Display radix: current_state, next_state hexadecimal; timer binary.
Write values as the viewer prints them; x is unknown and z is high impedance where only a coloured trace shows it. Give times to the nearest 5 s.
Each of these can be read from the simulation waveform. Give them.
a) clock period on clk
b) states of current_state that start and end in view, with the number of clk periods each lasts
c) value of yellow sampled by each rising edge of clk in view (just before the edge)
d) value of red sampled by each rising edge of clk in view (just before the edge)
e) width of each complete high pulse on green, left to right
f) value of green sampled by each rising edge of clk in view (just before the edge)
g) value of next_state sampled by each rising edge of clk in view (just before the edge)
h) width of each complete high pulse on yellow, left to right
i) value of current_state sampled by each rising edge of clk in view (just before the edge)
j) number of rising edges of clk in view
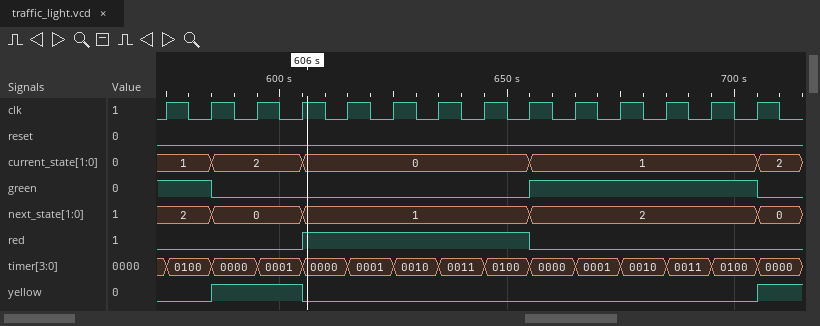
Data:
10 s
2: 2, 0: 5, 1: 5
0 0 1 1 0 0 0 0 0 0 0 0 0 0
0 0 0 0 1 1 1 1 1 0 0 0 0 0
50 s
1 1 0 0 0 0 0 0 0 1 1 1 1 1
2, 2, 0, 0, 1, 1, 1, 1, 1, 2, 2, 2, 2, 2
20 s
1, 1, 2, 2, 0, 0, 0, 0, 0, 1, 1, 1, 1, 1
14
